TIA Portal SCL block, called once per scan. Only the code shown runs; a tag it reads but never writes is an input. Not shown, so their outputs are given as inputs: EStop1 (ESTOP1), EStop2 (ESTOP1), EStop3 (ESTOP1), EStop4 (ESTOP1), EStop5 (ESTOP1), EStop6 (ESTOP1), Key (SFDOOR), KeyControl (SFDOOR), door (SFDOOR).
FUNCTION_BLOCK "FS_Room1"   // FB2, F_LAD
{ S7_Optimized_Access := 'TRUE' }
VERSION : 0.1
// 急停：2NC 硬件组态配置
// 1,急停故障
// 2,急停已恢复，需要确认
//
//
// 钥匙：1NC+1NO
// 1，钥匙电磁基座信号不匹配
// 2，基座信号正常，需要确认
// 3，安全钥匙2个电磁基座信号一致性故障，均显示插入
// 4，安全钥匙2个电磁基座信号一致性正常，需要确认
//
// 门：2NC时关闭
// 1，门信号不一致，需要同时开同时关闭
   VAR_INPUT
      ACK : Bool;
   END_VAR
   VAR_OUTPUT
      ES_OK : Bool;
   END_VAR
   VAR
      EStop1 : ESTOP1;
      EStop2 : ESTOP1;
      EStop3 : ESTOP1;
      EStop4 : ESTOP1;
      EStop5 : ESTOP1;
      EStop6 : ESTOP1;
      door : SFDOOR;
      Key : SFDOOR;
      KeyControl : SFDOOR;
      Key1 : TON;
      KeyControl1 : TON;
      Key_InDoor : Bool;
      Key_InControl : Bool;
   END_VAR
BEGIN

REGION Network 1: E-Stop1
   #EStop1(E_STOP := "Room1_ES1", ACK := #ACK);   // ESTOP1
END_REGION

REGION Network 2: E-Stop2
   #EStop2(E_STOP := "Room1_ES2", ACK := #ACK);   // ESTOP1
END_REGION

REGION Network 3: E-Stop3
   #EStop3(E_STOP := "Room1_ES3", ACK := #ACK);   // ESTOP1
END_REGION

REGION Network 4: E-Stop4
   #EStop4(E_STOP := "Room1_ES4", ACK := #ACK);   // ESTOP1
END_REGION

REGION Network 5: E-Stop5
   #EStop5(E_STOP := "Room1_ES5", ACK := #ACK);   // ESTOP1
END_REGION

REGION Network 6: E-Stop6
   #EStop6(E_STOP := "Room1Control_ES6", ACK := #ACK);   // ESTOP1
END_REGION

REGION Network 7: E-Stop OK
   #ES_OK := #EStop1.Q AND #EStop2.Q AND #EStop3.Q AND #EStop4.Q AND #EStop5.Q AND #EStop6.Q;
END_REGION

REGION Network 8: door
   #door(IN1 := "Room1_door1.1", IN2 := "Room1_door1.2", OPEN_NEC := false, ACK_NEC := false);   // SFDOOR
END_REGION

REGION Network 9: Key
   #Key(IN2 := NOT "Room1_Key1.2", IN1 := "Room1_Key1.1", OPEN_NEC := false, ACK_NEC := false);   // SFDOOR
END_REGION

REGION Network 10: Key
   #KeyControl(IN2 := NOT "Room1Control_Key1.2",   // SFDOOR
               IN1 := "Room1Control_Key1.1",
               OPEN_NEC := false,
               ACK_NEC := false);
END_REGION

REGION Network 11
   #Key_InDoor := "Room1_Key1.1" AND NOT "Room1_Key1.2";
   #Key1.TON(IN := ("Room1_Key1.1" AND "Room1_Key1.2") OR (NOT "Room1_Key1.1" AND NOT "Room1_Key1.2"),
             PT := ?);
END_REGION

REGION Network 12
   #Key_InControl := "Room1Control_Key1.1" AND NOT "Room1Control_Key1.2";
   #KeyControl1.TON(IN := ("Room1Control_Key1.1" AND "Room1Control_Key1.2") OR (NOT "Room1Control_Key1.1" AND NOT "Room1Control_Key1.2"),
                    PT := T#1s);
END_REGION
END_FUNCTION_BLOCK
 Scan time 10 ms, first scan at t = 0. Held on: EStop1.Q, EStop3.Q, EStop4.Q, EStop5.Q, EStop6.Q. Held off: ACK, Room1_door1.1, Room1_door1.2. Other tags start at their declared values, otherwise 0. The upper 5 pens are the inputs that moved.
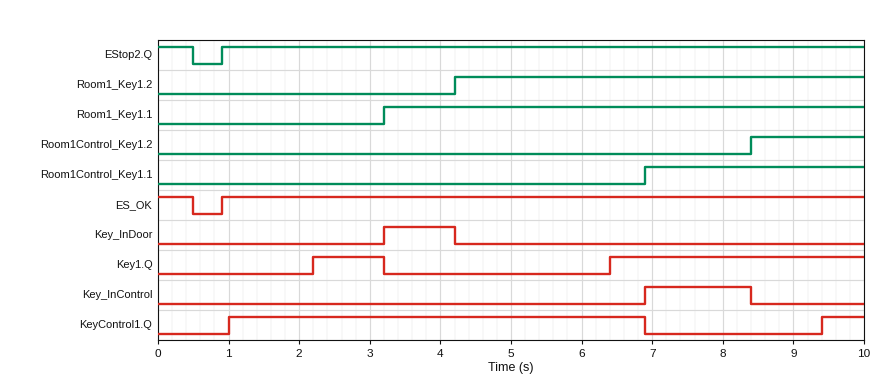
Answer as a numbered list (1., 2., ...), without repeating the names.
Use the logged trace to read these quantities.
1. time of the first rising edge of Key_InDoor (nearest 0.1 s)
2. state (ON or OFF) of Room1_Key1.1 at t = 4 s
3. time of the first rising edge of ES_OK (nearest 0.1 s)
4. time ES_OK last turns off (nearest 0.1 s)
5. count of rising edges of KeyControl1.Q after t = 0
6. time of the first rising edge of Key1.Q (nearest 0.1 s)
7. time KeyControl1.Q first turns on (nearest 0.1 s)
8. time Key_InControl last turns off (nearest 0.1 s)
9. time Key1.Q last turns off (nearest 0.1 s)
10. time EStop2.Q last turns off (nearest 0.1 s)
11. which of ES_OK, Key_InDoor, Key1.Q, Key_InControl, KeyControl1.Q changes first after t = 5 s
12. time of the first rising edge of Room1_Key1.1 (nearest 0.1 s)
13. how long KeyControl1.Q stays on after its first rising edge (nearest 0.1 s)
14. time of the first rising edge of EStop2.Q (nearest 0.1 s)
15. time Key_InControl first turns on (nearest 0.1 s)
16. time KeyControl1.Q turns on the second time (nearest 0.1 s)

1. 3.2 s
2. ON
3. 0.9 s
4. 0.5 s
5. 2
6. 2.2 s
7. 1.0 s
8. 8.4 s
9. 3.2 s
10. 0.5 s
11. Key1.Q
12. 3.2 s
13. 5.9 s
14. 0.9 s
15. 6.9 s
16. 9.4 s
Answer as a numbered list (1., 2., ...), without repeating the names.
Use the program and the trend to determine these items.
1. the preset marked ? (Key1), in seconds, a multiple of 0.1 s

1. 2.2 s
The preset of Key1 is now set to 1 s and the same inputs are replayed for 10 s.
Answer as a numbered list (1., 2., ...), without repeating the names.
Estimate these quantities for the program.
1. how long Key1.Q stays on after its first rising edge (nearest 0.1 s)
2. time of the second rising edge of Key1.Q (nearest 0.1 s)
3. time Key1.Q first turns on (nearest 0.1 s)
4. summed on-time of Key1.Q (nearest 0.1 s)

1. 2.2 s
2. 5.2 s
3. 1.0 s
4. 7.0 s
